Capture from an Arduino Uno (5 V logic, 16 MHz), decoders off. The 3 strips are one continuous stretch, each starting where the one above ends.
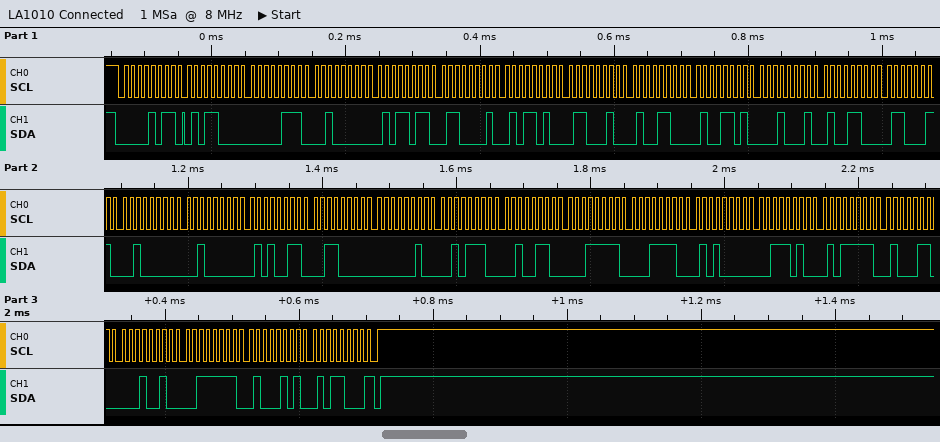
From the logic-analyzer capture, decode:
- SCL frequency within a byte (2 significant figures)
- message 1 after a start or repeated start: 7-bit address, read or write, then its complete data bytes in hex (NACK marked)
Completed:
100 kHz
0x05 read: 58 07 20 5B 61 5A 62 4C 4D 11 4C 63 20 20 53 30 02 2E 26 1F 1E 50 3A 5F 46 12 3F 45 58 NACK
